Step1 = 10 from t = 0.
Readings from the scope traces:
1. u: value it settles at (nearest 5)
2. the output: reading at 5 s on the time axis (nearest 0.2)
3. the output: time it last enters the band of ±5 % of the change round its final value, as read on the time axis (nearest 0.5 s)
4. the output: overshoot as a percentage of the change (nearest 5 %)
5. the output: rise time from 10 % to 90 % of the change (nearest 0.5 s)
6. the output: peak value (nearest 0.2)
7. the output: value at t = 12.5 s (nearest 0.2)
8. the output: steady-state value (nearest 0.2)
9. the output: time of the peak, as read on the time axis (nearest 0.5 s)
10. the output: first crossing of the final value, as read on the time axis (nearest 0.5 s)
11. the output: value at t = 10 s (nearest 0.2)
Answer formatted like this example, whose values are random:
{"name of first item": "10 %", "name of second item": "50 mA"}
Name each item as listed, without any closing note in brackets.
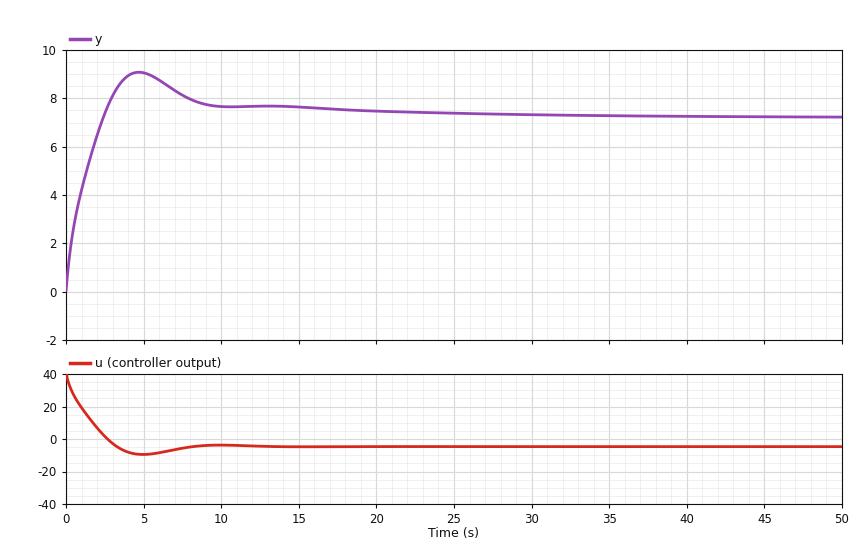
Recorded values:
{"u: value it settles at": "-5", "the output: reading at 5 s on the time axis": "9.0", "the output: time it last enters the band of ±5 % of the change round its final value, as read on the time axis": "17.0 s", "the output: overshoot as a percentage of the change": "25 %", "the output: rise time from 10 % to 90 % of the change": "2.0 s", "the output: peak value": "9.0", "the output: value at t = 12.5 s": "7.6", "the output: steady-state value": "7.2", "the output: time of the peak, as read on the time axis": "4.5 s", "the output: first crossing of the final value, as read on the time axis": "2.5 s", "the output: value at t = 10 s": "7.6"}
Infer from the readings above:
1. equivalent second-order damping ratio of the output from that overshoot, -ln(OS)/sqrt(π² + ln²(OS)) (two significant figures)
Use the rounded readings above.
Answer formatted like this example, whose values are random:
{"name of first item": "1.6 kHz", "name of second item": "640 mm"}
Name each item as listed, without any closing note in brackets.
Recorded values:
{"equivalent second-order damping ratio of the output from that overshoot, -ln(OS)/sqrt(π² + ln²(OS))": "0.40"}
